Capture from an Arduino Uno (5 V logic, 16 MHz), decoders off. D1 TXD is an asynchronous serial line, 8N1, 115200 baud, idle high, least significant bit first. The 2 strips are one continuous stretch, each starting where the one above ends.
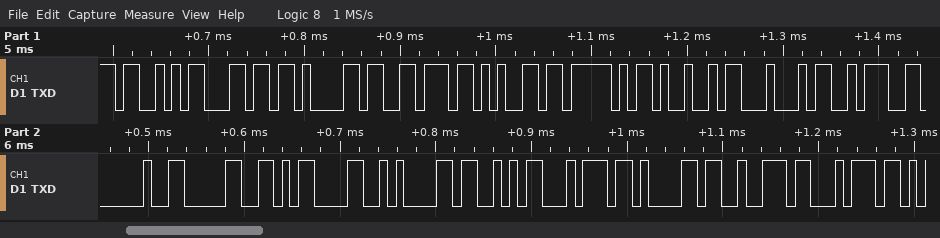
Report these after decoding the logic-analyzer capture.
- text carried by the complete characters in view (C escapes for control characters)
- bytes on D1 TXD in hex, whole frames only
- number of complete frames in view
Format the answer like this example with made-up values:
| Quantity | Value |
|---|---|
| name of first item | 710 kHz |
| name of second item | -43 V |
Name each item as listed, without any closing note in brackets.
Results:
| Quantity | Value |
|---|---|
| text carried by the complete characters in view | "Slave_ID: 0\r\nStart" |
| bytes on D1 TXD in hex, whole frames only | 0x53 0x6C 0x61 0x76 0x65 0x5F 0x49 0x44 0x3A 0x20 0x30 0x0D 0x0A 0x53 0x74 0x61 0x72 0x74 |
| number of complete frames in view | 18 |
